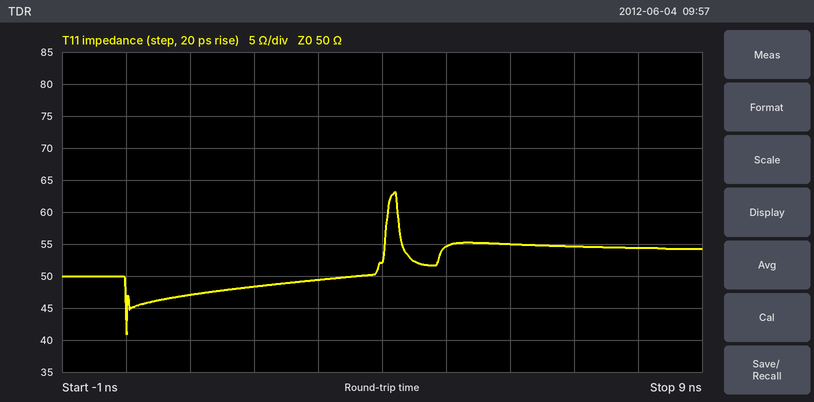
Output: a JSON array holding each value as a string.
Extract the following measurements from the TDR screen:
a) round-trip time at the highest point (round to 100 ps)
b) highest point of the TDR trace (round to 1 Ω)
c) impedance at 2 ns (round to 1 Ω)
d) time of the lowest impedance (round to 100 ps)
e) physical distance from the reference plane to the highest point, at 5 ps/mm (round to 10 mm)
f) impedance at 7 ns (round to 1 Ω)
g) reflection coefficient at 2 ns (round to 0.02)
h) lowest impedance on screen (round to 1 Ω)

["4.2 ns", "63 Ω", "48 Ω", "0.0 ns", "420 mm", "55 Ω", "-0.02", "41 Ω"]
